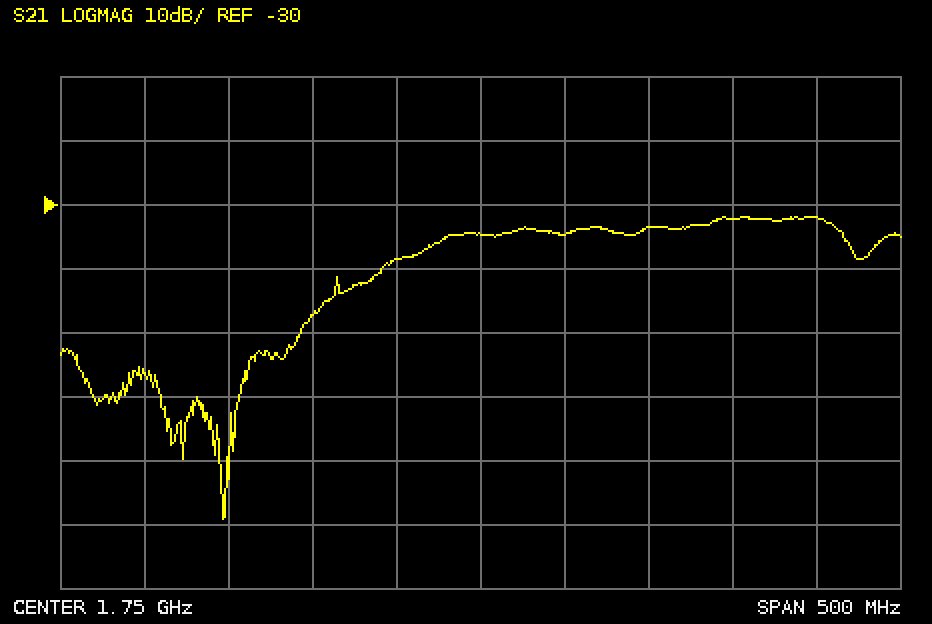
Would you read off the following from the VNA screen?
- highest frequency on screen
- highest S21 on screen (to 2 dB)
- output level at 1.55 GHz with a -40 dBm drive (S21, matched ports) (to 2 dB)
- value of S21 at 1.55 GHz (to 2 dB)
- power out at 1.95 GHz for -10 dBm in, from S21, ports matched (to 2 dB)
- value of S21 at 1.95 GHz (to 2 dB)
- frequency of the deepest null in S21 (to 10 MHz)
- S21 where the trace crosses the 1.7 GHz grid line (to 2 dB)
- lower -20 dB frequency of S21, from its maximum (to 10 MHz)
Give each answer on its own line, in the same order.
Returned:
2 GHz
-32 dB
-96 dBm
-56 dB
-42 dBm
-32 dB
1.60 GHz
-38 dB
1.64 GHz
